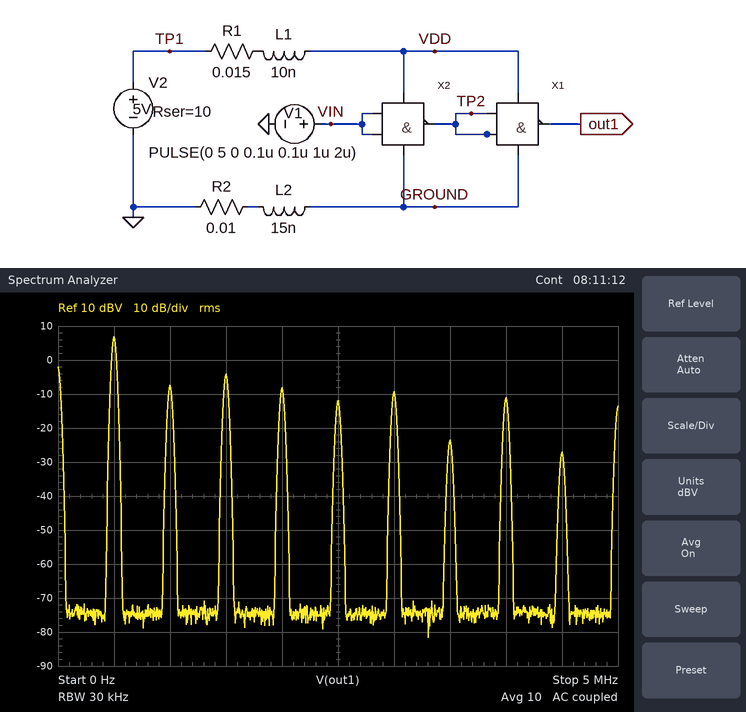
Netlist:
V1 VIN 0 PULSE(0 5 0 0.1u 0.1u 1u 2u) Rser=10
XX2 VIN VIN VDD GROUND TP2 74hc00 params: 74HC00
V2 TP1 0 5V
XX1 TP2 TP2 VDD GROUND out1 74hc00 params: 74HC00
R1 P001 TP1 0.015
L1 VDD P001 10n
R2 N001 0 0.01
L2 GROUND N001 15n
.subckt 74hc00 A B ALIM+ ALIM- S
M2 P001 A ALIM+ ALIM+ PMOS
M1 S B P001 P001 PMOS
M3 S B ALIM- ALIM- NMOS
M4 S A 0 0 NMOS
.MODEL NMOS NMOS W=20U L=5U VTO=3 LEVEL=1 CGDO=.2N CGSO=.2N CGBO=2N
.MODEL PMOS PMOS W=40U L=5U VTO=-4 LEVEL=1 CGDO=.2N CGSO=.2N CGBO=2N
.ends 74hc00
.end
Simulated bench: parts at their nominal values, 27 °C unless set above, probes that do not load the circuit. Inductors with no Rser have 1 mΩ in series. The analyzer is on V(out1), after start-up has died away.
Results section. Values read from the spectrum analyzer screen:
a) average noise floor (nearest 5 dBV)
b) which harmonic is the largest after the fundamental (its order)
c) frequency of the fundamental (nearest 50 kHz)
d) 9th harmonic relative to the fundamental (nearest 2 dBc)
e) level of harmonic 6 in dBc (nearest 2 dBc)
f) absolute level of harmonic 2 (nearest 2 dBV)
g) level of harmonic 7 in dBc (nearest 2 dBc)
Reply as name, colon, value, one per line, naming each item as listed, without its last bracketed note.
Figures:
average noise floor: -75 dBV
which harmonic is the largest after the fundamental: 3
frequency of the fundamental: 500 kHz
9th harmonic relative to the fundamental: -34 dBc
level of harmonic 6 in dBc: -16 dBc
absolute level of harmonic 2: -8 dBV
level of harmonic 7 in dBc: -30 dBc
